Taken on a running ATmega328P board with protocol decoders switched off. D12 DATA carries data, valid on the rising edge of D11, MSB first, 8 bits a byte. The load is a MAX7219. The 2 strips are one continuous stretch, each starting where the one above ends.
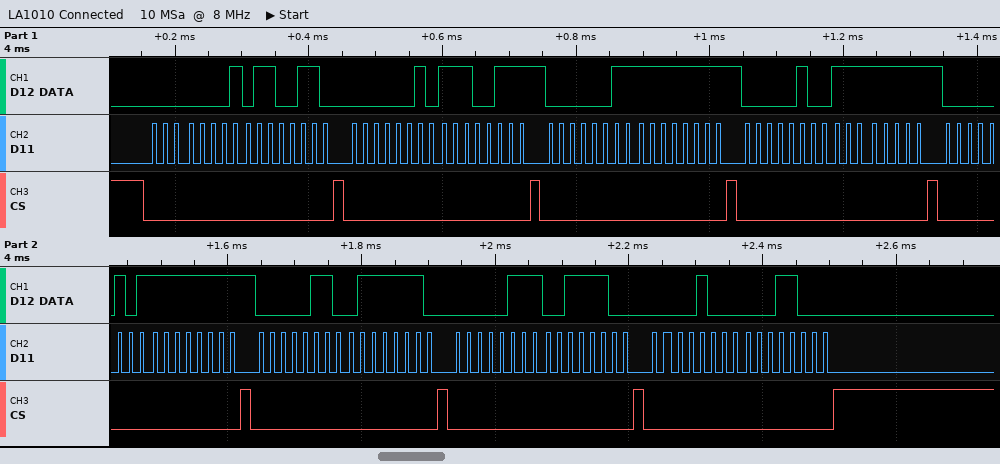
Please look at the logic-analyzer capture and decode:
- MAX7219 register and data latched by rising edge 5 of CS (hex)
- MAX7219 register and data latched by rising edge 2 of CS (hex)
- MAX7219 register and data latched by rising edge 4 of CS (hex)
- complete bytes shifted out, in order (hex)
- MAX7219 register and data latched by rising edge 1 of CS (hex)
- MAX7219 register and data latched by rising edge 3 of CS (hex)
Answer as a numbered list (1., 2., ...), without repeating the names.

1. register 0x5, data 0xFF
2. register 0x2, data 0xE7
3. register 0x4, data 0xFF
4. 0x01 0x66 0x02 0xE7 0x03 0xFF 0x04 0xFF 0x05 0xFF 0x06 0x7E 0x07 0x3C 0x08 0x18
5. register 0x1, data 0x66
6. register 0x3, data 0xFF
